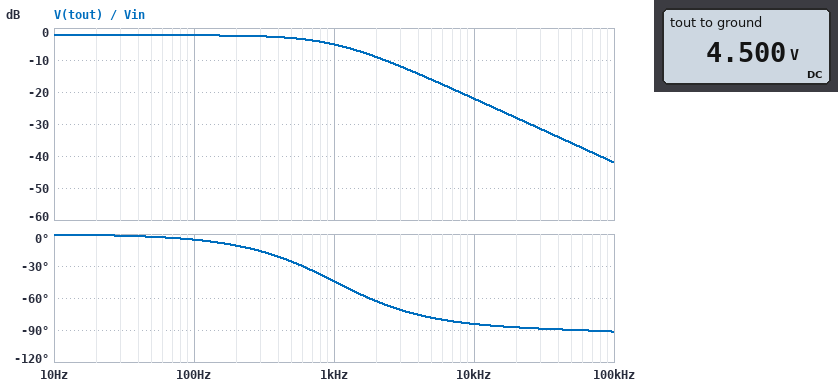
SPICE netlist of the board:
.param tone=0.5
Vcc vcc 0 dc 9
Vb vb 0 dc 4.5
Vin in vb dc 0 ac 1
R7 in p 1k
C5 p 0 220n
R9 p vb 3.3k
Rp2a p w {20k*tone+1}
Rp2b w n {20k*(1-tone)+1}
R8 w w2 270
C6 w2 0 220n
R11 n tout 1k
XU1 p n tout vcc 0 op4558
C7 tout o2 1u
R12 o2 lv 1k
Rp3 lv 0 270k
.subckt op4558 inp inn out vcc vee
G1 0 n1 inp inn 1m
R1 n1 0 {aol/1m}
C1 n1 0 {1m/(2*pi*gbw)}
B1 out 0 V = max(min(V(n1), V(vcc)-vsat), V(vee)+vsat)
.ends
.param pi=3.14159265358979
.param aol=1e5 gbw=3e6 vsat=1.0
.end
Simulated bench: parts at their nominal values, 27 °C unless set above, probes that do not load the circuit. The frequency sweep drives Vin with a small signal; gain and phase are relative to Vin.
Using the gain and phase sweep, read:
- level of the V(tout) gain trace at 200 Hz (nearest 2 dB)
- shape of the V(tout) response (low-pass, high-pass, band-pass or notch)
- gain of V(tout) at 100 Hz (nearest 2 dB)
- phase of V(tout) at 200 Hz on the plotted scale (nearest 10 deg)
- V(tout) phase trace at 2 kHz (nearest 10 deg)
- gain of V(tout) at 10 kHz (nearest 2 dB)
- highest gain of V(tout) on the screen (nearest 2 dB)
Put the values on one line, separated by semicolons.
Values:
-2 dB; low-pass; -2 dB; -10 deg; -60 deg; -22 dB; -2 dB
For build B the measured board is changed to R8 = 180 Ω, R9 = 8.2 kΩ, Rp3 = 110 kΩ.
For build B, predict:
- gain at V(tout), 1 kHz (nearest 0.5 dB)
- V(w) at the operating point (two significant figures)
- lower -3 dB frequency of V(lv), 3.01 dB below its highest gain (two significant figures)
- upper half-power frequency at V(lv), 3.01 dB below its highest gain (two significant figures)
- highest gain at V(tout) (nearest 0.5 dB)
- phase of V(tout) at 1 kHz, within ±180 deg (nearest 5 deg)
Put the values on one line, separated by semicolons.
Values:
-4.5 dB; 4.5 V; 1.4 Hz; 890 Hz; -1.0 dB; -50 deg
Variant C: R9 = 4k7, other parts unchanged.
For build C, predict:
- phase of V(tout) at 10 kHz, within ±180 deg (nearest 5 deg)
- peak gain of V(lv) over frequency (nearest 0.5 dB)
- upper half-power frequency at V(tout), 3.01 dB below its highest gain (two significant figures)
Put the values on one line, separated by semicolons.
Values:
-85 deg; -1.5 dB; 960 Hz
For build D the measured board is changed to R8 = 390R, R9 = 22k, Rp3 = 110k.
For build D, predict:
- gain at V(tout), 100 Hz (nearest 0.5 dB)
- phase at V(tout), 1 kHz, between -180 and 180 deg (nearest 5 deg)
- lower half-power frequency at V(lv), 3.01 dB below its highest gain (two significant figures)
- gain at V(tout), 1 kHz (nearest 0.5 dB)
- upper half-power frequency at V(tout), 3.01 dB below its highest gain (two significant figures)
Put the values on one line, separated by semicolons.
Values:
-0.5 dB; -50 deg; 1.4 Hz; -4.5 dB; 820 Hz
